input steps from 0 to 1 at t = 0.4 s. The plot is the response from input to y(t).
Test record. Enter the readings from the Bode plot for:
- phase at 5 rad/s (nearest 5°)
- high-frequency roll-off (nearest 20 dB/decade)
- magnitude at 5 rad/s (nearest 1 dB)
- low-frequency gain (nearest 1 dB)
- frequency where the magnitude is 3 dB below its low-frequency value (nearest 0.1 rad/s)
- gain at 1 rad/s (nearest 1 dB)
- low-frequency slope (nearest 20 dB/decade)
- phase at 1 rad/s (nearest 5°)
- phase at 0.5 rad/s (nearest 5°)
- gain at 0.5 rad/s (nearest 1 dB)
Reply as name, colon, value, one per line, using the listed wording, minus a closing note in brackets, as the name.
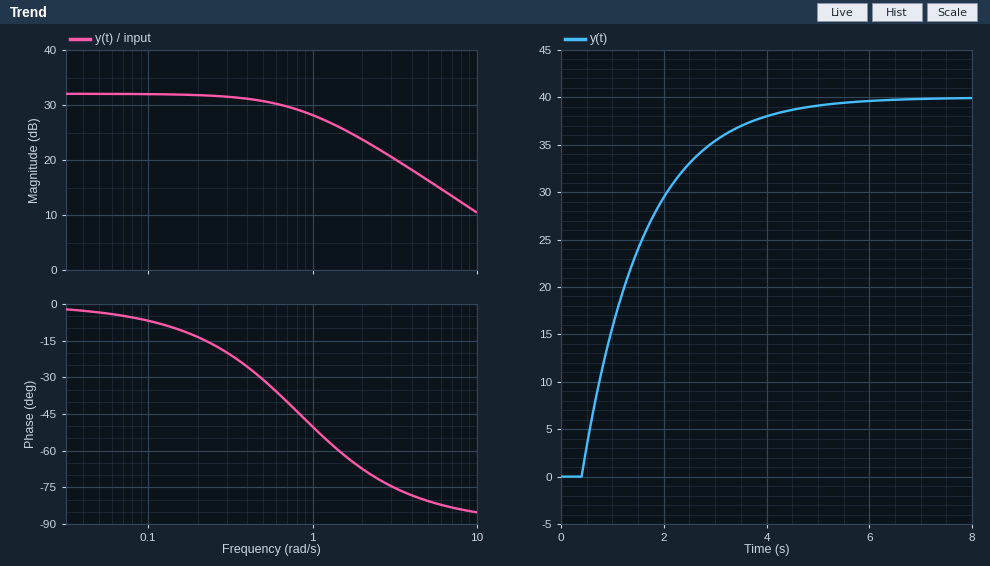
phase at 5 rad/s: -80°
high-frequency roll-off: -20 dB/decade
magnitude at 5 rad/s: 16 dB
low-frequency gain: 32 dB
frequency where the magnitude is 3 dB below its low-frequency value: 0.8 rad/s
gain at 1 rad/s: 28 dB
low-frequency slope: 0 dB/decade
phase at 1 rad/s: -50°
phase at 0.5 rad/s: -30°
gain at 0.5 rad/s: 31 dB
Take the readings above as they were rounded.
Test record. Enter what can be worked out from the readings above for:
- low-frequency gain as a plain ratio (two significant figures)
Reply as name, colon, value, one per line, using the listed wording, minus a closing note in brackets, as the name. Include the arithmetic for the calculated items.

low-frequency gain as a plain ratio: 10^(32 / 20) = 40
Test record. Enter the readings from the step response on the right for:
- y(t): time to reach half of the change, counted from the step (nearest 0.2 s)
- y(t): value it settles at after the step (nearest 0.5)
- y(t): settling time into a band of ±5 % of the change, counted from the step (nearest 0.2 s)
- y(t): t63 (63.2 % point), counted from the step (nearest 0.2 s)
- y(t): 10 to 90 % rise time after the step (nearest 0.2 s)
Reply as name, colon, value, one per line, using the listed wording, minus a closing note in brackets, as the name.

y(t): time to reach half of the change, counted from the step: 0.8 s
y(t): value it settles at after the step: 40.0
y(t): settling time into a band of ±5 % of the change, counted from the step: 3.6 s
y(t): t63 (63.2 % point), counted from the step: 1.2 s
y(t): 10 to 90 % rise time after the step: 2.6 s
